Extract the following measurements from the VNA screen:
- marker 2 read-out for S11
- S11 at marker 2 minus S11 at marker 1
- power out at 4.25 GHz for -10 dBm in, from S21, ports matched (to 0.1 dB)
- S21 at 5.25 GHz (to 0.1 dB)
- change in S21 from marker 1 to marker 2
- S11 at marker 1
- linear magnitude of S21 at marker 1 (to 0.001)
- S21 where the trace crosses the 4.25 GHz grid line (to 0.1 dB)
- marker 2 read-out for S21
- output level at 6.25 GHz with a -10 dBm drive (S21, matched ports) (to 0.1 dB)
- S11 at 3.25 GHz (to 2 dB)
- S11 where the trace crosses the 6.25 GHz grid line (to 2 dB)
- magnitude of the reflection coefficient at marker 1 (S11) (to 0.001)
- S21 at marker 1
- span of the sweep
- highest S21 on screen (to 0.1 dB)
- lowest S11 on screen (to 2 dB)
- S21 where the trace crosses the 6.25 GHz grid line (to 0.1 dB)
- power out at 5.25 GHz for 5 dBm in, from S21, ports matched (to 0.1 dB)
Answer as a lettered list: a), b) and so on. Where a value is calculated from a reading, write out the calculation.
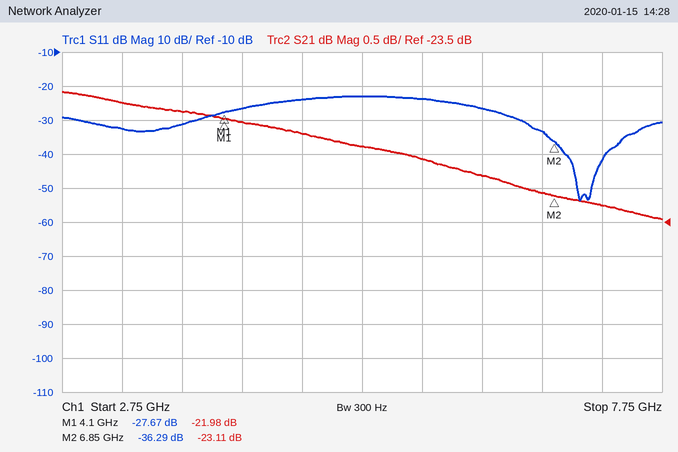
a) -36.29 dB
b) -36.29 − (-27.67) = -8.62 dB
c) -10 dBm + (-22.0 dB) = -32.0 dBm
d) -22.4 dB
e) -23.11 − (-21.98) = -1.13 dB
f) -27.67 dB
g) 10^(-21.98/20) ≈ 0.080
h) -22.0 dB
i) -23.11 dB
j) -10 dBm + (-22.8 dB) = -32.8 dBm
k) -32 dB
l) -26 dB
m) 10^(-27.67/20) ≈ 0.041
n) -21.98 dB
o) 5 GHz
p) -21.6 dB
q) -54 dB
r) -22.8 dB
s) 5 dBm + (-22.4 dB) = -17.4 dBm
